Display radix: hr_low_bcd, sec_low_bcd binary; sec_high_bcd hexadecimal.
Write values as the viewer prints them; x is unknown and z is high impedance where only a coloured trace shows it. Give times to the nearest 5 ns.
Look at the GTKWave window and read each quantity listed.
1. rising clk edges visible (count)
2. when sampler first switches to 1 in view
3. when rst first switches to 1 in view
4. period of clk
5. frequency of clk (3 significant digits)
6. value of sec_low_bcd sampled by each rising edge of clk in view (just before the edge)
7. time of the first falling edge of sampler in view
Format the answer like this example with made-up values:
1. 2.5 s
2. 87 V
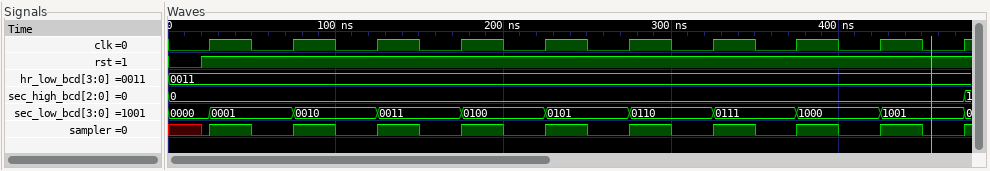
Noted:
1. 10
2. 25 ns
3. 20 ns
4. 50 ns
5. 20.0 MHz
6. 0000, 0001, 0010, 0011, 0100, 0101, 0110, 0111, 1000, 1001
7. 50 ns
